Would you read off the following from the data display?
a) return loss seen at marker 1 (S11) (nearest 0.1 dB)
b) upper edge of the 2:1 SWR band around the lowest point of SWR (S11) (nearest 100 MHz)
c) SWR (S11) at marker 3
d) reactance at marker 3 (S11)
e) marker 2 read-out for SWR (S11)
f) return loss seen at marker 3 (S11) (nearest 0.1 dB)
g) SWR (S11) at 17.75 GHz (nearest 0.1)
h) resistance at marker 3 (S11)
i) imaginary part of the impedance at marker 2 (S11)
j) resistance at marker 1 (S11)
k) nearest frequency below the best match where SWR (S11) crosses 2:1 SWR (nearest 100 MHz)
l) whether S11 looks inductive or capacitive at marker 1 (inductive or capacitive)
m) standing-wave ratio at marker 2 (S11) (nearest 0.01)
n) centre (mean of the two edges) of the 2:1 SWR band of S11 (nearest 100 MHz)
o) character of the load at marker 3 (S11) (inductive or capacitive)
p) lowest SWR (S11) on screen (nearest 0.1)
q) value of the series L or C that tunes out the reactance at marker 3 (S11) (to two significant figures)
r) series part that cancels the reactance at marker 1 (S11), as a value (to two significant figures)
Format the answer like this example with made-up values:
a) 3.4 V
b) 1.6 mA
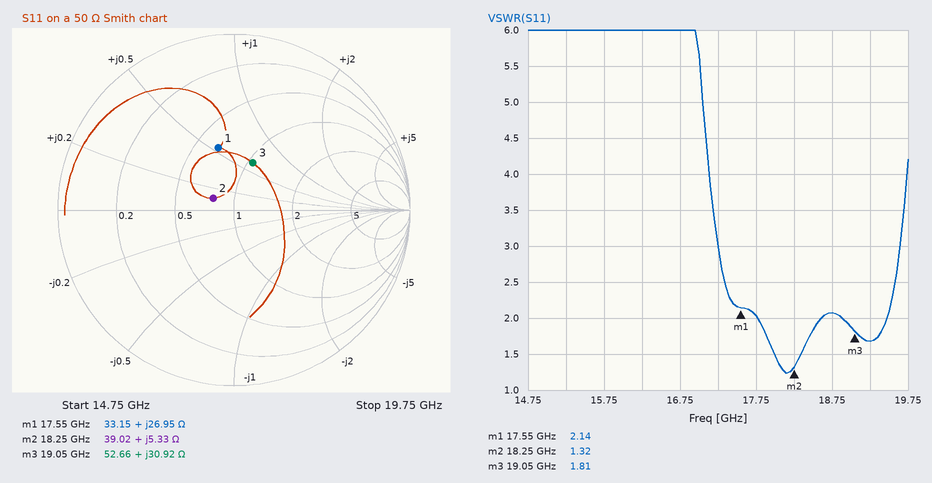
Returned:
a) 8.8 dB
b) 18.6 GHz
c) 1.81
d) +30.92 Ω
e) 1.32
f) 10.8 dB
g) 2.0
h) 52.66 Ω
i) +5.33 Ω
j) 33.15 Ω
k) 17.8 GHz
l) inductive
m) 1.32
n) 18.2 GHz
o) inductive
p) 1.2
q) 270 fF
r) 340 fF
